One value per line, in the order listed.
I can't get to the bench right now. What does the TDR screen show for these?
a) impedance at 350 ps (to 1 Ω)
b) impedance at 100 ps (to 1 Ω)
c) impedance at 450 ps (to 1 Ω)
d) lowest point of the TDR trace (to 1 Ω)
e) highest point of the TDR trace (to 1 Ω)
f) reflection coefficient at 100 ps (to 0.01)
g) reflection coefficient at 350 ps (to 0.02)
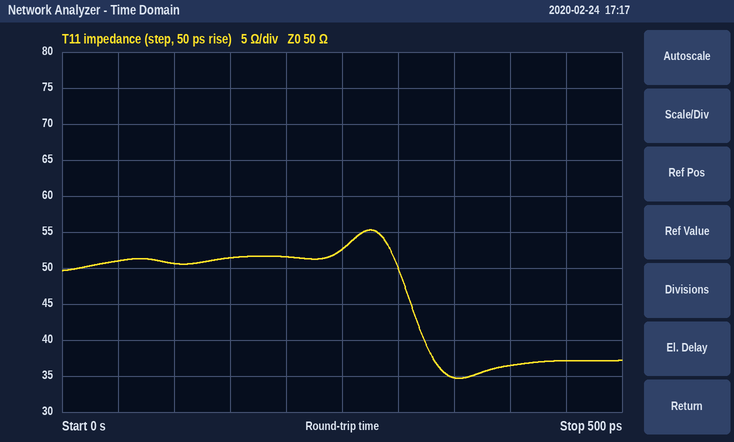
35 Ω
51 Ω
37 Ω
35 Ω
55 Ω
+0.01
-0.18
